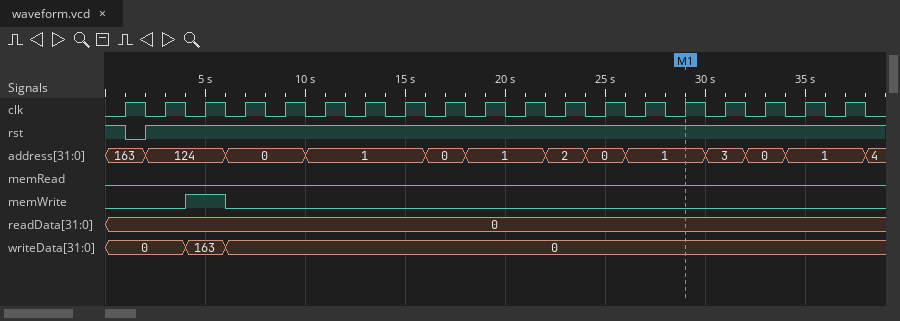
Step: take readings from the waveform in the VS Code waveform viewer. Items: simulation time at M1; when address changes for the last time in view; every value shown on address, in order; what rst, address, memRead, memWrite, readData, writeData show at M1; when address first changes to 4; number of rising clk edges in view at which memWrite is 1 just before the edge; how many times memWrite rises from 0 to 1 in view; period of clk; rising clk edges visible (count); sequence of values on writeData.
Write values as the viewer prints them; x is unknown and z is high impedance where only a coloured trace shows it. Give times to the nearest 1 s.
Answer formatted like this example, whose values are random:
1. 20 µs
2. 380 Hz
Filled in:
1. 29 s
2. 38 s
3. 163, 124, 0, 1, 0, 1, 2, 0, 1, 3, 0, 1, 4
4. rst=1, address=1, memRead=0, memWrite=0, readData=0, writeData=0
5. 38 s
6. 1
7. 1
8. 2 s
9. 19
10. 0, 163, 0
